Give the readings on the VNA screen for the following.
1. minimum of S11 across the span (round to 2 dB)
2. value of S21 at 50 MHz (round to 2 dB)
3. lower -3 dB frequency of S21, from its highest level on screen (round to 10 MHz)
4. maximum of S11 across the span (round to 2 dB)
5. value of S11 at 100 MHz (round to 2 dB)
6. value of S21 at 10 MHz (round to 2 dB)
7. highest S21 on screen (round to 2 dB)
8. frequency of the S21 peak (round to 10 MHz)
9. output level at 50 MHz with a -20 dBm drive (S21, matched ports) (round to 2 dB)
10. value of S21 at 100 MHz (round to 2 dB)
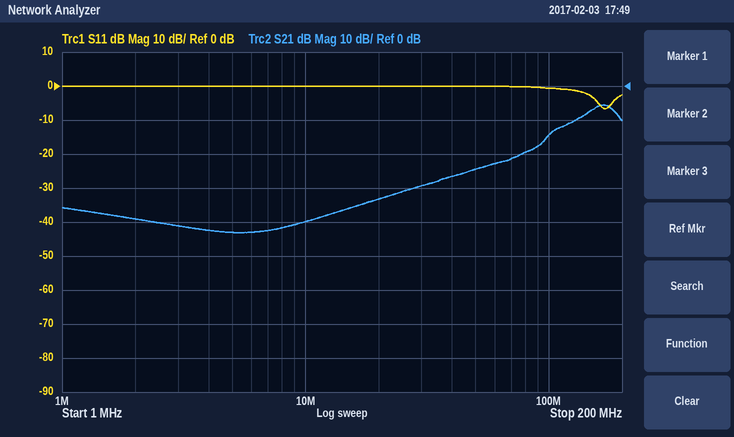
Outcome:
-6 dB
-24 dB
140 MHz
0 dB
0 dB
-40 dB
-6 dB
170 MHz
-44 dBm
-14 dB
